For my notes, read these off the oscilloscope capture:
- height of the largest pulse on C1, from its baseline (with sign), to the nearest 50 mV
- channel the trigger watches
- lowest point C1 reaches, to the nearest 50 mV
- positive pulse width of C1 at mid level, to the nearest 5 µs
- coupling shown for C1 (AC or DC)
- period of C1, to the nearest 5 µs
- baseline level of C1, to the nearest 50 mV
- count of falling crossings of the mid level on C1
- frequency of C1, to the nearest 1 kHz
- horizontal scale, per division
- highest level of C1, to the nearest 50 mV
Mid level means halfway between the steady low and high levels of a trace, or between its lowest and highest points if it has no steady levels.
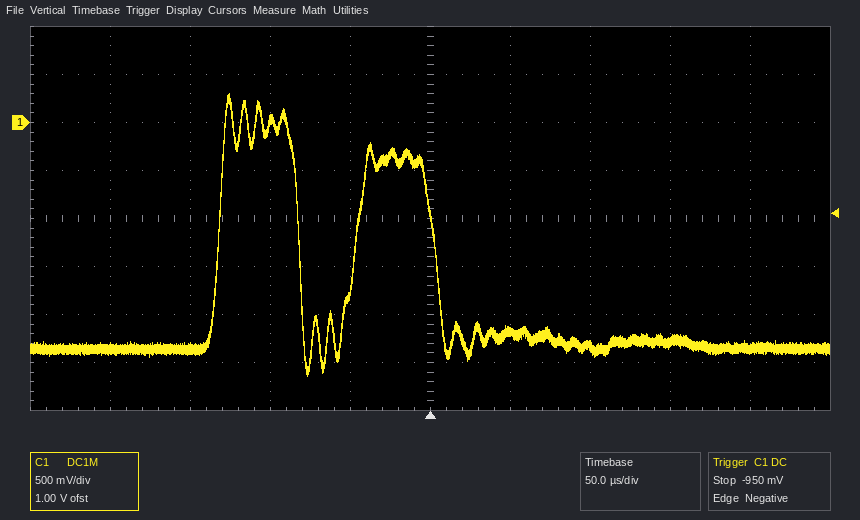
+2.65 V
C1
-2.65 V
50 µs
DC
85 µs
-2.35 V
2
12 kHz
50 µs
300 mV
